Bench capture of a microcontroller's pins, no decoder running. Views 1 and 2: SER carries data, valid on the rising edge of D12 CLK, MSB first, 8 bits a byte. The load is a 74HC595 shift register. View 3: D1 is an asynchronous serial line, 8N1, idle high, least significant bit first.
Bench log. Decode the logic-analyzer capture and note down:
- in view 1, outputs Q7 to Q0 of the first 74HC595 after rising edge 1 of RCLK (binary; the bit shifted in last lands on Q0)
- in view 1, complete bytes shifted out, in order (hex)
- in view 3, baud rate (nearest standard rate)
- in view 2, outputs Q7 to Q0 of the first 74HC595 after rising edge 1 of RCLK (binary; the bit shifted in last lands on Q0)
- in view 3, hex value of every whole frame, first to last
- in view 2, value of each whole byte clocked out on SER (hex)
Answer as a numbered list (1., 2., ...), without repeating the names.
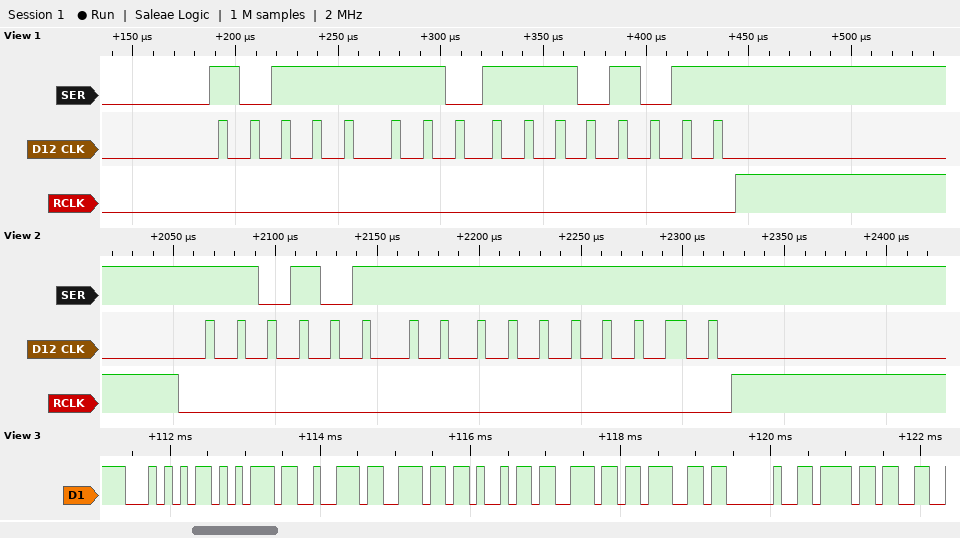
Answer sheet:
1. 11101011
2. BE EB
3. 9600 baud
4. 11111111
5. 54 75 72 6E 69 6E 67 20 6F
6. 0xD7 0xFF
